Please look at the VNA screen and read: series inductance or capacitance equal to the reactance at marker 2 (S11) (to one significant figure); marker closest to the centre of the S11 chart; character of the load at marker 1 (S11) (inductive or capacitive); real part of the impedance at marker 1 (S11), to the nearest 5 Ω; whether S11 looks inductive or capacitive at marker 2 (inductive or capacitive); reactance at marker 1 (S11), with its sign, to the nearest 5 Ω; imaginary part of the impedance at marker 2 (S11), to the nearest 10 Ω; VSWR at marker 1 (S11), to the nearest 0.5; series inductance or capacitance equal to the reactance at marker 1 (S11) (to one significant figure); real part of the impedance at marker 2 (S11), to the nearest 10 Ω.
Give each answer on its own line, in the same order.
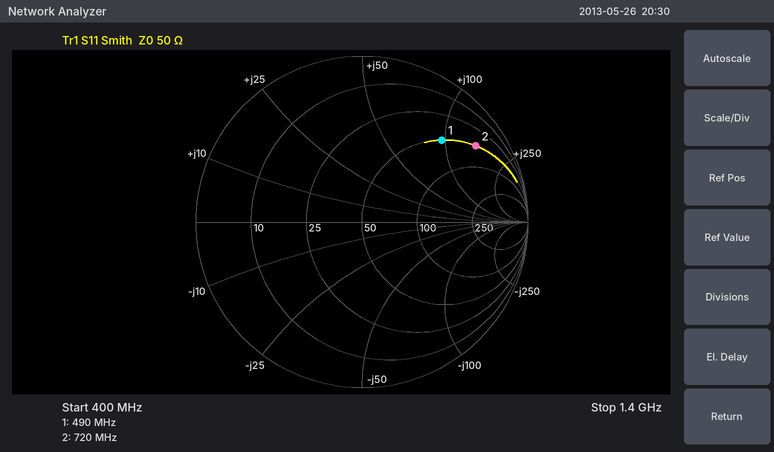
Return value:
30 nH
marker 1
inductive
50 Ω
inductive
+95 Ω
+150 Ω
5.5
30 nH
50 Ω
